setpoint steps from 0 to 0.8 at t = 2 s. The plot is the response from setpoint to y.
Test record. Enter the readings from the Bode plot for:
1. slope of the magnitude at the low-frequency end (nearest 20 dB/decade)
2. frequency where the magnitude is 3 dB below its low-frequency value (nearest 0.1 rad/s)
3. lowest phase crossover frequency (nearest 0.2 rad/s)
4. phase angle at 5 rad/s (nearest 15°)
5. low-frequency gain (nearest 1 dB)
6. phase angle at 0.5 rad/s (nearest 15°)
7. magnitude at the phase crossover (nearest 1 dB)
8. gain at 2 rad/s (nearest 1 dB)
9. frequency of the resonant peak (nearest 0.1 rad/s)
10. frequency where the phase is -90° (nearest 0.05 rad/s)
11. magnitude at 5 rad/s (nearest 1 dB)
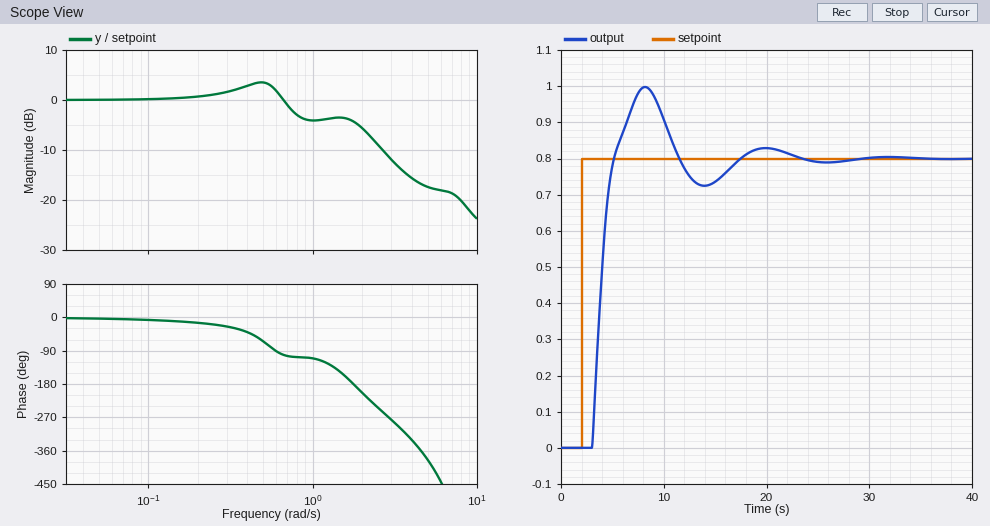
0 dB/decade
0.8 rad/s
1.8 rad/s
-390°
0 dB
-60°
-4 dB
-6 dB
0.5 rad/s
0.60 rad/s
-17 dB
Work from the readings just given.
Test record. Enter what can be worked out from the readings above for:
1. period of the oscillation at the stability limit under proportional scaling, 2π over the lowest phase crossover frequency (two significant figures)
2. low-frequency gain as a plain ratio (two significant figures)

3.5 s
1.0
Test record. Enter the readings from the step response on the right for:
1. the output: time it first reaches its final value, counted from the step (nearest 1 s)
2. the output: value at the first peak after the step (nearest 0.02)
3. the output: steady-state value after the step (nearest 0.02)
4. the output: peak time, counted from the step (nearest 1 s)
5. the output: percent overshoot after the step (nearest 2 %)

3 s
1.00
0.80
6 s
24 %
